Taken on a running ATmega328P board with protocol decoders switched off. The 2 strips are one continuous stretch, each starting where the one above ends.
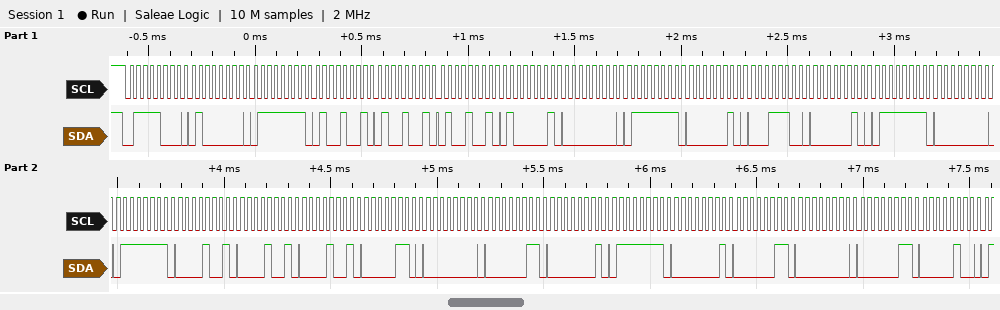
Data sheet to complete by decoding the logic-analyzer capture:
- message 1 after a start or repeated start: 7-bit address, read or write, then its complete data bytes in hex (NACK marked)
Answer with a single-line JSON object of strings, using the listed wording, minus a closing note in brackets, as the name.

{"message 1 after a start or repeated start: 7-bit address, read or write, then its complete data bytes in hex": "0x3C write: 40 7F 49 49 49 41 00 7F 02 1C 02 7F 00 7F 09 09 09 06 00 03 01 7F 01 03 00 03 04"}
